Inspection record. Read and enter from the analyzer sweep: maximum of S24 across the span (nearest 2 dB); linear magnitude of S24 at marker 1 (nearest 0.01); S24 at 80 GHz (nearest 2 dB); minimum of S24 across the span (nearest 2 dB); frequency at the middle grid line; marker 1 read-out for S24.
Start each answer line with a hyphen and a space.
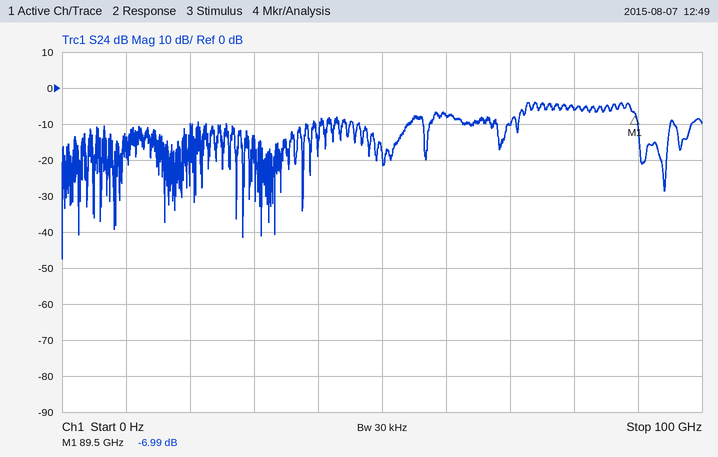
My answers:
- -4 dB
- 0.45
- -6 dB
- -48 dB
- 50 GHz
- -6.99 dB
